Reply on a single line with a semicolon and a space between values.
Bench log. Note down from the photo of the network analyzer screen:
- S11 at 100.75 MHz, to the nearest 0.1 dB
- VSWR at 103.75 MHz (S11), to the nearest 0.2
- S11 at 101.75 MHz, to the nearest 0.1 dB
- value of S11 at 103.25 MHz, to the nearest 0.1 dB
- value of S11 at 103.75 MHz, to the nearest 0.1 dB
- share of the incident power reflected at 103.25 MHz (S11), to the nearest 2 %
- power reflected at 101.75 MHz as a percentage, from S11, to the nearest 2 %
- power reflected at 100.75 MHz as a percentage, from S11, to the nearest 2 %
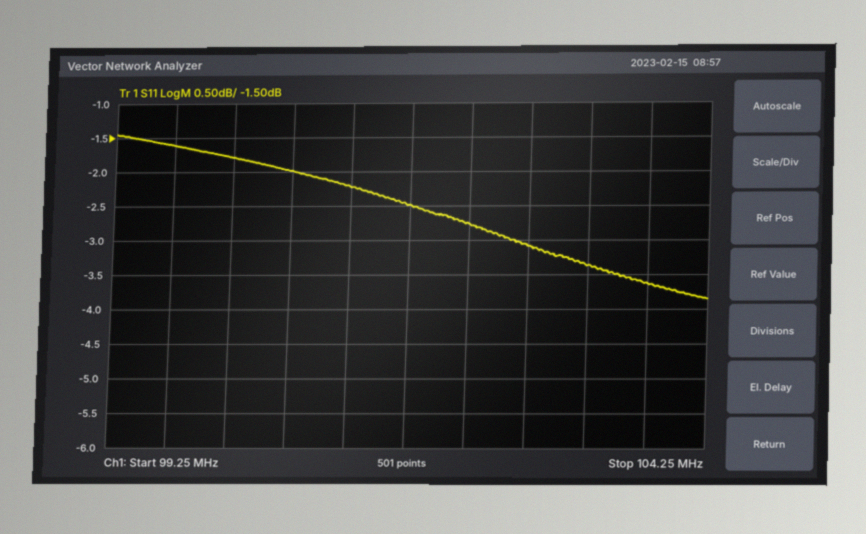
-2.0 dB; 4.8; -2.5 dB; -3.4 dB; -3.6 dB; 46 %; 56 %; 64 %
